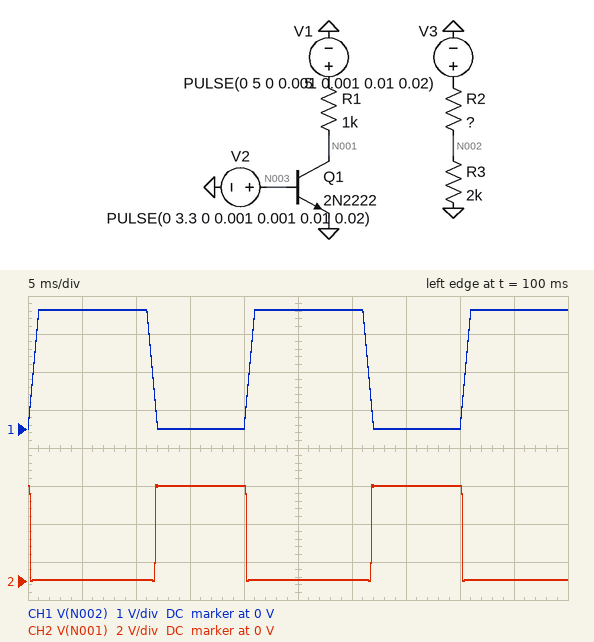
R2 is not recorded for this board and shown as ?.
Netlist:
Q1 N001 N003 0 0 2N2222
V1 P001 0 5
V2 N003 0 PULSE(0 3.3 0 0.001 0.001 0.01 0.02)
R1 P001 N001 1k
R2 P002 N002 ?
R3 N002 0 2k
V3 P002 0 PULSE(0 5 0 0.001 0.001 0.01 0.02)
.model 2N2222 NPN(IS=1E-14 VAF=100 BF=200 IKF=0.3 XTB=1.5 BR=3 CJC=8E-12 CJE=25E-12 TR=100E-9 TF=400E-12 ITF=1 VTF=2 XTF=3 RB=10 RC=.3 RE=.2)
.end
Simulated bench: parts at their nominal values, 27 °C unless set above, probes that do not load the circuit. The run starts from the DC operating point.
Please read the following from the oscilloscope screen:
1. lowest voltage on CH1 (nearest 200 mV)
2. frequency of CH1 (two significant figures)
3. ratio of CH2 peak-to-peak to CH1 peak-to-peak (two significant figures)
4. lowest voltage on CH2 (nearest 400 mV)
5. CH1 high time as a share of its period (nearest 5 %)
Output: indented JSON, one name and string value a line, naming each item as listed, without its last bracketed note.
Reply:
{
  "lowest voltage on CH1": "0 V",
  "frequency of CH1": "50 Hz",
  "ratio of CH2 peak-to-peak to CH1 peak-to-peak": "1.6",
  "lowest voltage on CH2": "0 V",
  "CH1 high time as a share of its period": "55 %"
}
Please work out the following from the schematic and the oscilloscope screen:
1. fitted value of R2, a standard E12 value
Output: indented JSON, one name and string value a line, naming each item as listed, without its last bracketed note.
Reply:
{
  "fitted value of R2, a standard E12 value": "1.2 kΩ"
}
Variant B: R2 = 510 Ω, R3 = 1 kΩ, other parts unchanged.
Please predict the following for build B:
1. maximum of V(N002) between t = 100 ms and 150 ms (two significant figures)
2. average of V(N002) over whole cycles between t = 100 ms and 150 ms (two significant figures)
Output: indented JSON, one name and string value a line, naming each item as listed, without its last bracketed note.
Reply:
{
  "maximum of V(N002) between t = 100 ms and 150 ms": "3.3 V",
  "average of V(N002) over whole cycles between t = 100 ms and 150 ms": "1.8 V"
}
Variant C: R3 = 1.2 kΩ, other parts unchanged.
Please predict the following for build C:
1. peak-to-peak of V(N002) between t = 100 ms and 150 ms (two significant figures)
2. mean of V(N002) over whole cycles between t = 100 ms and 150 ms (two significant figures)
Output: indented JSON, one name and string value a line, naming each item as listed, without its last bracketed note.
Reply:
{
  "peak-to-peak of V(N002) between t = 100 ms and 150 ms": "2.5 V",
  "mean of V(N002) over whole cycles between t = 100 ms and 150 ms": "1.4 V"
}
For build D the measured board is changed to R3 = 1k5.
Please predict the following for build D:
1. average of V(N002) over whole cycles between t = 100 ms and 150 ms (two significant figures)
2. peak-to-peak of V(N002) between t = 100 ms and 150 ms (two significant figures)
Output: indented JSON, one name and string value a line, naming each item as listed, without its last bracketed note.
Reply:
{
  "average of V(N002) over whole cycles between t = 100 ms and 150 ms": "1.5 V",
  "peak-to-peak of V(N002) between t = 100 ms and 150 ms": "2.8 V"
}
